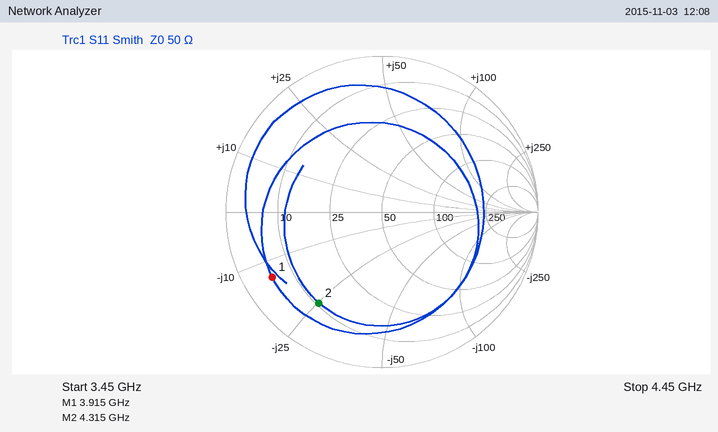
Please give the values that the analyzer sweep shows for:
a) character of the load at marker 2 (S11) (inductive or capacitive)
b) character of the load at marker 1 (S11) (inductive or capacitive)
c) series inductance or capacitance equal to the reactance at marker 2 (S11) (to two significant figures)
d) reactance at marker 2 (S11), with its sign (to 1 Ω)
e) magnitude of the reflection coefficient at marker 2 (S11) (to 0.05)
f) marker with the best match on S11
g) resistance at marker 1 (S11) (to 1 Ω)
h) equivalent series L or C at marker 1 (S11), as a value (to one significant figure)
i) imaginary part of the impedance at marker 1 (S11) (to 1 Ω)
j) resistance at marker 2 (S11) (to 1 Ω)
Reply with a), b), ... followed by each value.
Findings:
a) capacitive
b) capacitive
c) 1.5 pF
d) -25 Ω
e) 0.70
f) marker 2
g) 5 Ω
h) 3 pF
i) -14 Ω
j) 11 Ω
